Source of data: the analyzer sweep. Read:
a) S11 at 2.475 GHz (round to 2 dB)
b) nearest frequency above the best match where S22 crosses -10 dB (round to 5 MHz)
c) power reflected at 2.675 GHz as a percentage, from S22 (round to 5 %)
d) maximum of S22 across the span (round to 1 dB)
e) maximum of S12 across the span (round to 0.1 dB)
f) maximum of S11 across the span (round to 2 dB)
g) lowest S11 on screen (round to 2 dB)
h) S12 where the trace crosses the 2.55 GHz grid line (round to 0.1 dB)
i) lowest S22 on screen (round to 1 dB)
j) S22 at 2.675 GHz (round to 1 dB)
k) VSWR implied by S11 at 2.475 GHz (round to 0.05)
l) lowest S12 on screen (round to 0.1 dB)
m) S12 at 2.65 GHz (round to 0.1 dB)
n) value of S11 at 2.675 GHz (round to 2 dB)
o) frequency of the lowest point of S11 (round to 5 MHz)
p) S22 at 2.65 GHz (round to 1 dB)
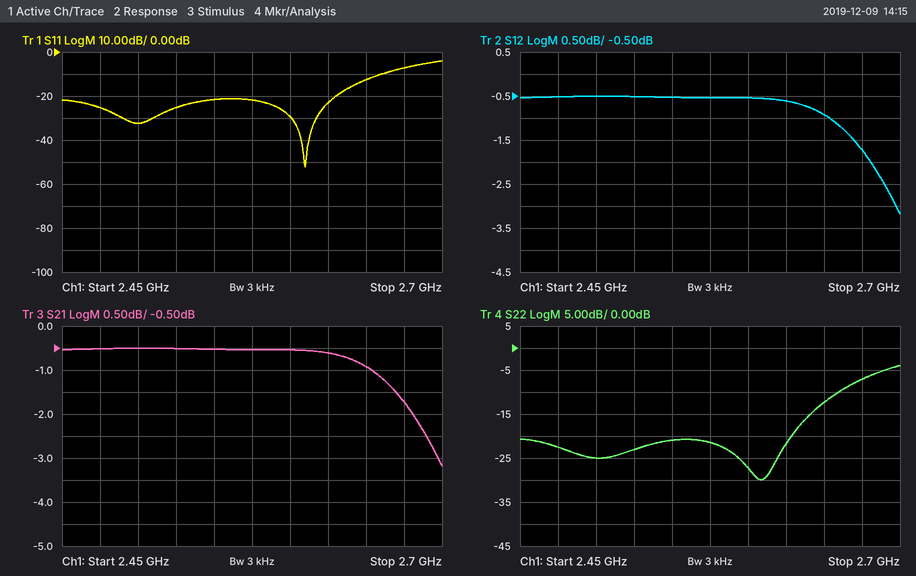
-26 dB
2.660 GHz
20 %
-4 dB
-0.5 dB
-4 dB
-52 dB
-0.5 dB
-30 dB
-7 dB
1.10
-3.2 dB
-0.9 dB
-8 dB
2.610 GHz
-12 dB
